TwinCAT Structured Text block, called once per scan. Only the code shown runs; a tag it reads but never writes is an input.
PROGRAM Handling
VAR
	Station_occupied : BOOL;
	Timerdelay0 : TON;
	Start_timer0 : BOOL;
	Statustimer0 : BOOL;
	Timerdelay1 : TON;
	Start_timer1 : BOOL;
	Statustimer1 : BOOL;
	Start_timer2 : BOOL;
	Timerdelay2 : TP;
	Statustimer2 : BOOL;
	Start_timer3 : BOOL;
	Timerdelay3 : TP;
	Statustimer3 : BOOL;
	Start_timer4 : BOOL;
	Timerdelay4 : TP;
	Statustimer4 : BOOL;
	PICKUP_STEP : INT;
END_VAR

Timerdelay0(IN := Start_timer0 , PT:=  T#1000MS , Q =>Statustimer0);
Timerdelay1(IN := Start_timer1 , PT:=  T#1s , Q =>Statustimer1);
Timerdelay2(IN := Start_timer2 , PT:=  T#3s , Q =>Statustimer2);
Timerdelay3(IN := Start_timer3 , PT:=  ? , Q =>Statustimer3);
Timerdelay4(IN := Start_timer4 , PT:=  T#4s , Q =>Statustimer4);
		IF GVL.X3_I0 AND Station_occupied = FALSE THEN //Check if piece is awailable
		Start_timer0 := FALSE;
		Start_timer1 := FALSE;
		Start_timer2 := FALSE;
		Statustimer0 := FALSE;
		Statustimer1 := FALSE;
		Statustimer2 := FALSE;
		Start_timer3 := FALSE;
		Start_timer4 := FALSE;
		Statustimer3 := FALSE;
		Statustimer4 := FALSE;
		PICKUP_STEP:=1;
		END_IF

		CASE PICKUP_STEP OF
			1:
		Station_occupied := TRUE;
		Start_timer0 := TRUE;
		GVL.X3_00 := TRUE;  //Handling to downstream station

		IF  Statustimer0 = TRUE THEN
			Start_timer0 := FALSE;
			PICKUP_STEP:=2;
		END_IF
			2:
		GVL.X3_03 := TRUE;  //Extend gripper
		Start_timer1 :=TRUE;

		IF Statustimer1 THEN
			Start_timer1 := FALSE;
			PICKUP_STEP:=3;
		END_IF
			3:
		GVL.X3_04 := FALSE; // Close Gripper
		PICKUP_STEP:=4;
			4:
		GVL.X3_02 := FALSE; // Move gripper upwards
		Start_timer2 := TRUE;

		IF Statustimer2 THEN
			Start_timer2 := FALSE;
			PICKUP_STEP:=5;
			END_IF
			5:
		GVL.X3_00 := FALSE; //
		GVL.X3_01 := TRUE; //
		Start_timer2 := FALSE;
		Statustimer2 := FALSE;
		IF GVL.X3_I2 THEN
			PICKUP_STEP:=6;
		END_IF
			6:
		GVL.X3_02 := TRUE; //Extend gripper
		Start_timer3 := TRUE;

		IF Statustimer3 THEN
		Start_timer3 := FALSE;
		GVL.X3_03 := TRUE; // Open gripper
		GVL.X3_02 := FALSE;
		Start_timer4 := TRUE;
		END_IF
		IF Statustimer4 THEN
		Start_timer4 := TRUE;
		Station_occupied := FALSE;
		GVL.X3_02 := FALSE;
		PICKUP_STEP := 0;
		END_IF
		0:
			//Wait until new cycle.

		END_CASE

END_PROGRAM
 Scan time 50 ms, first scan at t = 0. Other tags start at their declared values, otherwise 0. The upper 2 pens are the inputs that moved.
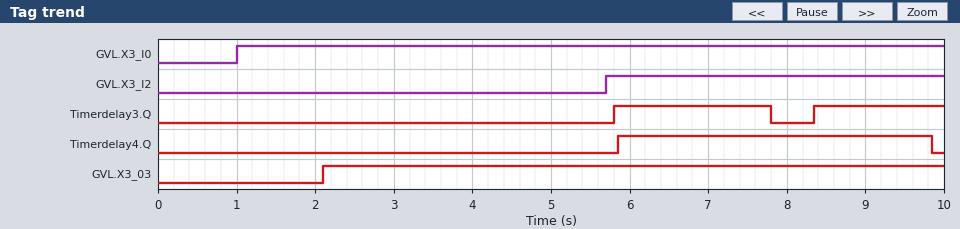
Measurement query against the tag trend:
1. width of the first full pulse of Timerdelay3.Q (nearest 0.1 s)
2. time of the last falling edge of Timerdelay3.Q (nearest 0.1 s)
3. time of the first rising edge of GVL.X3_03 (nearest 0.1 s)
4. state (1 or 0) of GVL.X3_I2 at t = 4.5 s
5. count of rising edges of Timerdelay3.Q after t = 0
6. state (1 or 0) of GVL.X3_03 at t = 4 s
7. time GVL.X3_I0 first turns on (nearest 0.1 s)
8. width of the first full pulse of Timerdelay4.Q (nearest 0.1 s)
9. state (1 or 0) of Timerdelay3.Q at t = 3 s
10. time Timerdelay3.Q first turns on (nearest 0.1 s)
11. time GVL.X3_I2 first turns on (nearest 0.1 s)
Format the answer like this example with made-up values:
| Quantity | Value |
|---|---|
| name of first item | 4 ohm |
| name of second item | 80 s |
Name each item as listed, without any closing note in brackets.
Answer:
| Quantity | Value |
|---|---|
| width of the first full pulse of Timerdelay3.Q | 2.0 s |
| time of the last falling edge of Timerdelay3.Q | 7.8 s |
| time of the first rising edge of GVL.X3_03 | 2.1 s |
| state (1 or 0) of GVL.X3_I2 at t = 4.5 s | 0 |
| count of rising edges of Timerdelay3.Q after t = 0 | 2 |
| state (1 or 0) of GVL.X3_03 at t = 4 s | 1 |
| time GVL.X3_I0 first turns on | 1.0 s |
| width of the first full pulse of Timerdelay4.Q | 4.0 s |
| state (1 or 0) of Timerdelay3.Q at t = 3 s | 0 |
| time Timerdelay3.Q first turns on | 5.8 s |
| time GVL.X3_I2 first turns on | 5.7 s |
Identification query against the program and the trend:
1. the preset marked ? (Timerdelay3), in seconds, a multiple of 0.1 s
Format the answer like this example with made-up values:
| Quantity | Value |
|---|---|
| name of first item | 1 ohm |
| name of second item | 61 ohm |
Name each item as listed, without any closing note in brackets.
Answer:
| Quantity | Value |
|---|---|
| the preset marked ? (Timerdelay3), in seconds, a multiple of 0.1 s | 2.0 s |
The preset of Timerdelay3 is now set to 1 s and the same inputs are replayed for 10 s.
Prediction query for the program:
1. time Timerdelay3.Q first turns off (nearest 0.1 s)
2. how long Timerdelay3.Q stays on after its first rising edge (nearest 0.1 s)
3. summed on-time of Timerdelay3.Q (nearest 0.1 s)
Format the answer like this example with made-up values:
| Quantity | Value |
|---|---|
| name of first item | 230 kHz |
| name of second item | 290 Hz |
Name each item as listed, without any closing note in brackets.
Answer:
| Quantity | Value |
|---|---|
| time Timerdelay3.Q first turns off | 6.8 s |
| how long Timerdelay3.Q stays on after its first rising edge | 1.0 s |
| summed on-time of Timerdelay3.Q | 2.0 s |
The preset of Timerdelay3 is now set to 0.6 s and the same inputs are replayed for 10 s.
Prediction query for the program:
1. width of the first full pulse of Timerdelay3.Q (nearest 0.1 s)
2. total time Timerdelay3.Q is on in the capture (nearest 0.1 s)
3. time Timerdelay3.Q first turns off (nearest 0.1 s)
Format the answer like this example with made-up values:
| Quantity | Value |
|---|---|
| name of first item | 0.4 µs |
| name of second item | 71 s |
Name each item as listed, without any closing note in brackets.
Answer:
| Quantity | Value |
|---|---|
| width of the first full pulse of Timerdelay3.Q | 0.6 s |
| total time Timerdelay3.Q is on in the capture | 1.2 s |
| time Timerdelay3.Q first turns off | 6.4 s |
